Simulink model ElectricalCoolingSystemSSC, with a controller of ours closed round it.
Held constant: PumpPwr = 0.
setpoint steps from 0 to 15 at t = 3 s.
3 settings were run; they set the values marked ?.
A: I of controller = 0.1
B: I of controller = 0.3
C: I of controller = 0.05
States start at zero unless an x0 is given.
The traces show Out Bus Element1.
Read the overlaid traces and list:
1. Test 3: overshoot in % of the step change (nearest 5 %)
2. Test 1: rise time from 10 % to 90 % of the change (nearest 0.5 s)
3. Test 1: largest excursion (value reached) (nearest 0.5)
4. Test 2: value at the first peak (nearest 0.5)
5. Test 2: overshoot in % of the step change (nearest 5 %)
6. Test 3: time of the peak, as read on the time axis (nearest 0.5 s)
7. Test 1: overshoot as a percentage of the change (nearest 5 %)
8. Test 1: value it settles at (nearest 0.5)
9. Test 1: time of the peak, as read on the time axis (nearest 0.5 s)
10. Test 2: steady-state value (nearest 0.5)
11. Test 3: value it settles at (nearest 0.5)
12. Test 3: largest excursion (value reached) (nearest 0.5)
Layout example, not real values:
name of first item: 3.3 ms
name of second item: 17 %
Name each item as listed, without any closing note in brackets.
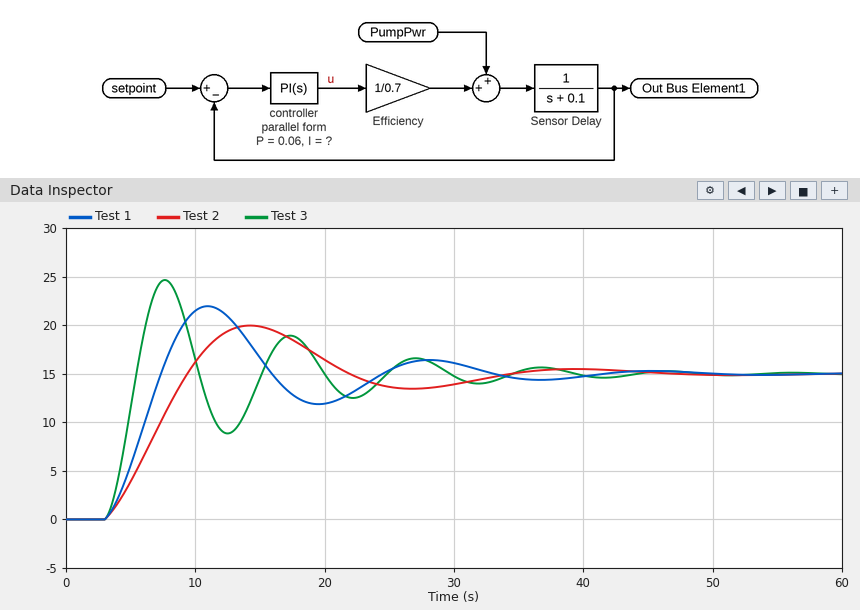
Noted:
Test 3: overshoot in % of the step change: 65 %
Test 1: rise time from 10 % to 90 % of the change: 3.0 s
Test 1: largest excursion (value reached): 22.0
Test 2: value at the first peak: 20.0
Test 2: overshoot in % of the step change: 35 %
Test 3: time of the peak, as read on the time axis: 7.5 s
Test 1: overshoot as a percentage of the change: 45 %
Test 1: value it settles at: 15.0
Test 1: time of the peak, as read on the time axis: 11.0 s
Test 2: steady-state value: 15.0
Test 3: value it settles at: 15.0
Test 3: largest excursion (value reached): 24.5
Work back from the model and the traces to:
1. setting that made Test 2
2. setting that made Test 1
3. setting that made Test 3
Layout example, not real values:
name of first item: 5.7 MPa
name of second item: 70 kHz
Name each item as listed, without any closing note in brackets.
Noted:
setting that made Test 2: C
setting that made Test 1: A
setting that made Test 3: B
